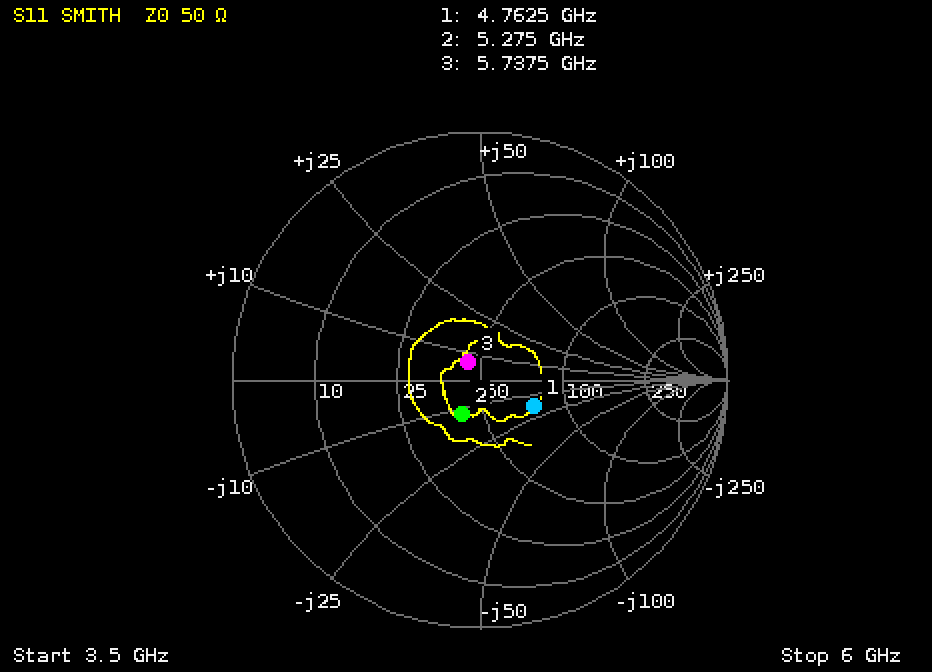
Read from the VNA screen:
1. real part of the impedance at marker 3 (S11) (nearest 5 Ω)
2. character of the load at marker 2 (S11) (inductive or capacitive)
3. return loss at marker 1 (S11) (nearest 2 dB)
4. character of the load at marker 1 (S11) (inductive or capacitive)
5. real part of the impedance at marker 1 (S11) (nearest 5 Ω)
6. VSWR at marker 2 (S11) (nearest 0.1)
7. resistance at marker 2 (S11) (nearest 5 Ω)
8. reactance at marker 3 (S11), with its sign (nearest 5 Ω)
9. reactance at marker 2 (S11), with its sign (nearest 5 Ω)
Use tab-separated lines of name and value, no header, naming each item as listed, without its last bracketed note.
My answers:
real part of the impedance at marker 3 (S11)	45 Ω
character of the load at marker 2 (S11)	capacitive
return loss at marker 1 (S11)	12 dB
character of the load at marker 1 (S11)	capacitive
real part of the impedance at marker 1 (S11)	75 Ω
VSWR at marker 2 (S11)	1.4
resistance at marker 2 (S11)	40 Ω
reactance at marker 3 (S11), with its sign	+5 Ω
reactance at marker 2 (S11), with its sign	-10 Ω
